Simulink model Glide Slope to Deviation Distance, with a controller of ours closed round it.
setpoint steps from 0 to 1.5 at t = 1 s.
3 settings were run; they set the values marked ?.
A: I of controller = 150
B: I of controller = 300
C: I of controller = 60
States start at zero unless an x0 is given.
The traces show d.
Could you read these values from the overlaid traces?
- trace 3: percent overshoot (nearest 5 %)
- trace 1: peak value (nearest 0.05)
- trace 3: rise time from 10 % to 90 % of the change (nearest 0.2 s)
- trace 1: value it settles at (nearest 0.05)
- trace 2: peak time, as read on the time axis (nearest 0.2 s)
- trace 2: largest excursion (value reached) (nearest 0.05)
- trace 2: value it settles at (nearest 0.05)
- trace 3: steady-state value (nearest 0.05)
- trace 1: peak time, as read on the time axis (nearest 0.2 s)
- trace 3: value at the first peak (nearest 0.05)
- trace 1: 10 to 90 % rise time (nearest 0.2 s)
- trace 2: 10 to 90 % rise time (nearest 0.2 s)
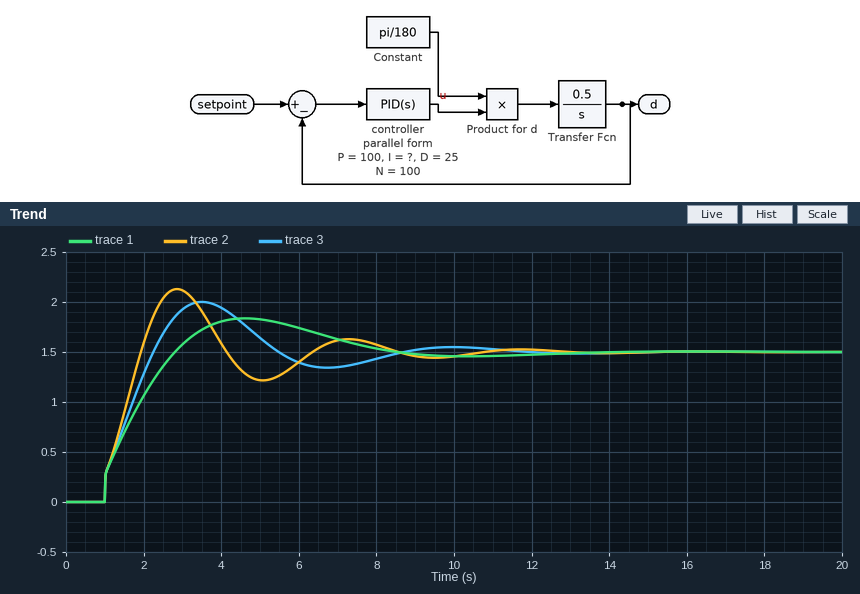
35 %
1.85
1.0 s
1.50
2.8 s
2.15
1.50
1.50
4.6 s
2.00
1.4 s
0.8 s
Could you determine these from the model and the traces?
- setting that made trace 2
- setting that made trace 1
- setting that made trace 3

B
C
A
